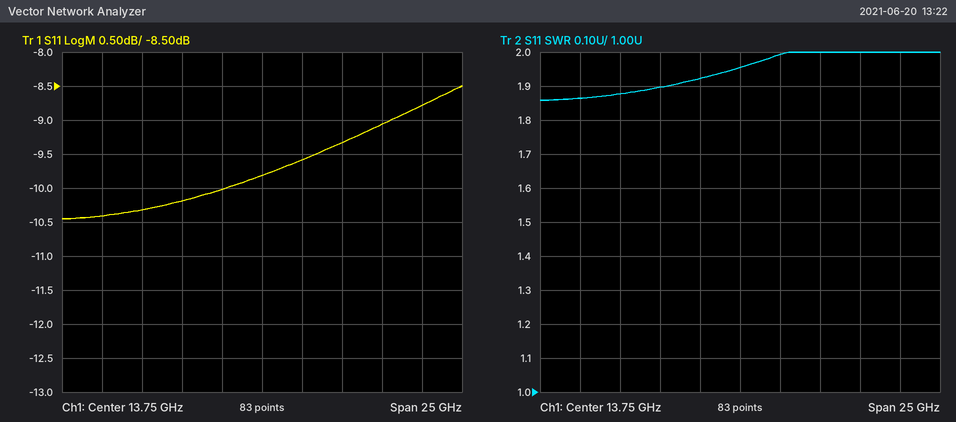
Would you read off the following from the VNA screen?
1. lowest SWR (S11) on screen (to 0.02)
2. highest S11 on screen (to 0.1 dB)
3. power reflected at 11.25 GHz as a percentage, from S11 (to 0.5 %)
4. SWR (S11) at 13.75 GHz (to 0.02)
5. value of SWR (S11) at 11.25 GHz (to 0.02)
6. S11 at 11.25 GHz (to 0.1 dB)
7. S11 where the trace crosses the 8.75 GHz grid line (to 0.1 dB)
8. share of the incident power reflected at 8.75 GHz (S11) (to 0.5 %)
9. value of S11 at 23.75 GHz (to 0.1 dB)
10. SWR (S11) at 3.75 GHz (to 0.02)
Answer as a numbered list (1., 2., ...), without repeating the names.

1. 1.86
2. -8.5 dB
3. 10.0 %
4. 1.96
5. 1.92
6. -10.0 dB
7. -10.2 dB
8. 9.5 %
9. -8.8 dB
10. 1.86
